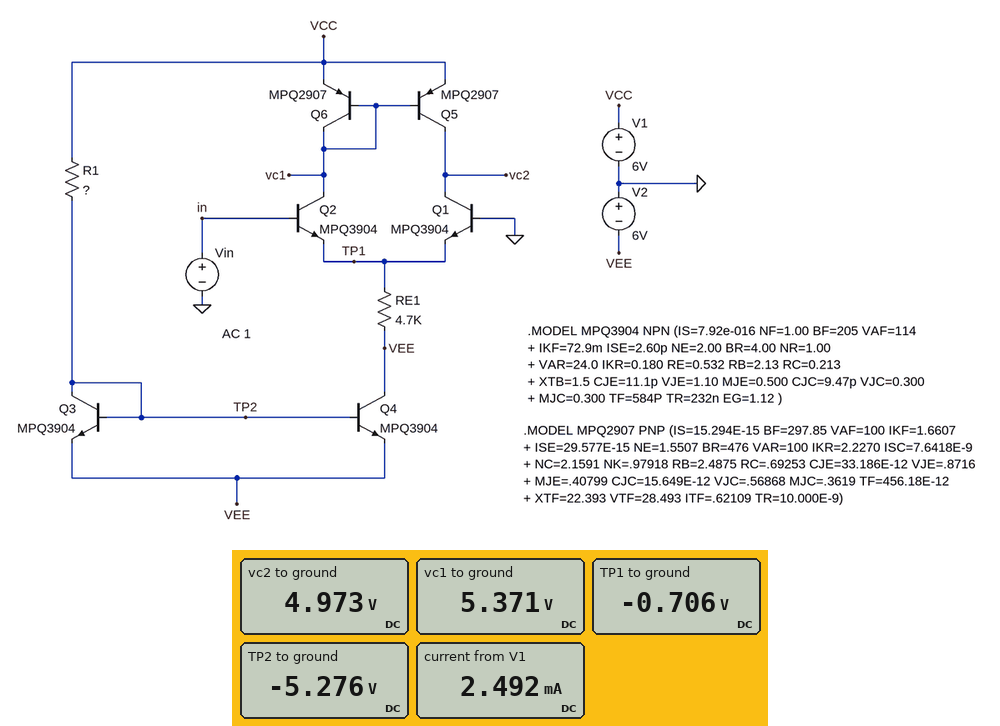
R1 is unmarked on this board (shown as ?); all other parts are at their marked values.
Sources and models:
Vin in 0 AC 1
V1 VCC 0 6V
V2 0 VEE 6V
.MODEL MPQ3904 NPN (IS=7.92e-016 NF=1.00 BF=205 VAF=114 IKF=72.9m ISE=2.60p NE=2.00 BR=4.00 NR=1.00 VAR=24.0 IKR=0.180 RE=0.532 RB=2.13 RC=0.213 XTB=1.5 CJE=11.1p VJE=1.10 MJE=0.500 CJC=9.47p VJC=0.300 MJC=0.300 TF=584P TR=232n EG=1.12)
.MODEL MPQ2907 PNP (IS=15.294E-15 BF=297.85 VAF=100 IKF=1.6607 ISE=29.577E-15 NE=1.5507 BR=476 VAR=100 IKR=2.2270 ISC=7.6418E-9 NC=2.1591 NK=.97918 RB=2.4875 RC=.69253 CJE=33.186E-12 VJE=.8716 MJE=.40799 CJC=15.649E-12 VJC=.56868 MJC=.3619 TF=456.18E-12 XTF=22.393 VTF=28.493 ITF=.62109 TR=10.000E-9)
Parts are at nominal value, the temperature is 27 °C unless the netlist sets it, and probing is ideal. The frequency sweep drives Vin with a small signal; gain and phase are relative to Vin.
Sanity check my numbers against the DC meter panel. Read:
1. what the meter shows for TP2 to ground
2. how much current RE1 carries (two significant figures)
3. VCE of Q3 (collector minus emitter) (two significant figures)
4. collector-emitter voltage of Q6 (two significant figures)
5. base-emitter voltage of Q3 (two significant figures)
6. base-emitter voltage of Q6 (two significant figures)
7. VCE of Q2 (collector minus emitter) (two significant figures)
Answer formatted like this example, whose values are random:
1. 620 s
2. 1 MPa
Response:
1. -5.276 V
2. 1.1 mA
3. 720 mV
4. -630 mV
5. 720 mV
6. -630 mV
7. 6.1 V
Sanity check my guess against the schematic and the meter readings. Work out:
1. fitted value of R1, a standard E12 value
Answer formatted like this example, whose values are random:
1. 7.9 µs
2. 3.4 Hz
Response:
1. 8.2 kΩ
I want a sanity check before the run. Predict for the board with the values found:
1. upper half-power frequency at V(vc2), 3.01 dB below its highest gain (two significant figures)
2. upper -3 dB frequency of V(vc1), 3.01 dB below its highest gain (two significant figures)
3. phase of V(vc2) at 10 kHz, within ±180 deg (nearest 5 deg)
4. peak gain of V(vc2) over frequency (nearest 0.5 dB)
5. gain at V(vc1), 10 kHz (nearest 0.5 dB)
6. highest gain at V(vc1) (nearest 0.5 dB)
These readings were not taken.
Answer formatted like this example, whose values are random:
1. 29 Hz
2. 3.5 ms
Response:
1. 54 kHz
2. 59 kHz
3. -10 deg
4. 66.0 dB
5. -11.5 dB
6. -11.5 dB
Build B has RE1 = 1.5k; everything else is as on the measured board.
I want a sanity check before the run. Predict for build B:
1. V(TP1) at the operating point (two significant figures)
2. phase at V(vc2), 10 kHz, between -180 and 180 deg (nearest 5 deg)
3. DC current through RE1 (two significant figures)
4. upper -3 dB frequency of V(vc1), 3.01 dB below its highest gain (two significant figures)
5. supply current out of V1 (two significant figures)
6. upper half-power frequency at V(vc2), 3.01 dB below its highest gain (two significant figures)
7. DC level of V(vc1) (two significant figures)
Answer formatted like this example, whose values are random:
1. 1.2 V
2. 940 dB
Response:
1. -740 mV
2. -5 deg
3. 3.5 mA
4. 180 kHz
5. 4.9 mA
6. 160 kHz
7. 5.3 V
